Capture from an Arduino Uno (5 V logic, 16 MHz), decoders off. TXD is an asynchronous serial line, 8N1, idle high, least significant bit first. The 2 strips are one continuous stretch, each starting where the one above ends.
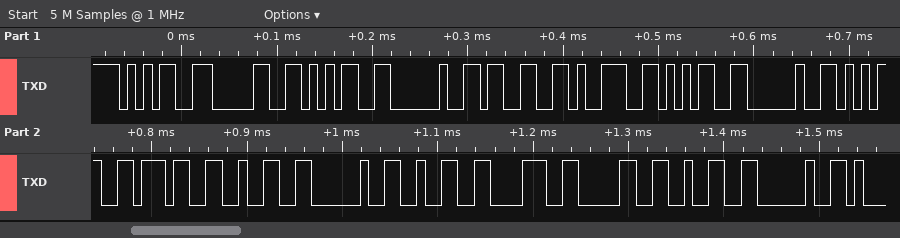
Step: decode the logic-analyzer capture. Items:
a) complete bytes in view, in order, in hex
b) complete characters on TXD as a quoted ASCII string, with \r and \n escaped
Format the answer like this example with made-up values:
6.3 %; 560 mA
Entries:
0x35 0x30 0x35 0x20 0x33 0x39 0x35 0x20 0x35 0x37 0x32 0x20 0x32 0x38 0x30 0x32 0x20; "505 395 572 2802 "
